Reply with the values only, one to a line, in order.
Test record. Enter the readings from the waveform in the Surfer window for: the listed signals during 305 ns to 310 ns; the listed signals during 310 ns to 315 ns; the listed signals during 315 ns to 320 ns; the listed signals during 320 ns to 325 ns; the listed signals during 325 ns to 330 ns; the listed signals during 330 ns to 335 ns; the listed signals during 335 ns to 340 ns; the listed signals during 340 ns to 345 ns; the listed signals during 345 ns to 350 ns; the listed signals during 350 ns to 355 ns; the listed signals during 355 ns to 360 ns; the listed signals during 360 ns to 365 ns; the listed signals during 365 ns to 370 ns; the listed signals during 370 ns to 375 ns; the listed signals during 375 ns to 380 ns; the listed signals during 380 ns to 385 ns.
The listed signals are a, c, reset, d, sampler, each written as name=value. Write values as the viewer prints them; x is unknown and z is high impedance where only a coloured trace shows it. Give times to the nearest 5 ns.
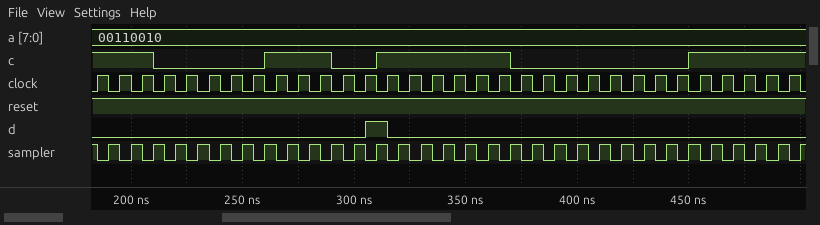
a=00110010, c=0, reset=1, d=1, sampler=0
a=00110010, c=1, reset=1, d=1, sampler=1
a=00110010, c=1, reset=1, d=0, sampler=0
a=00110010, c=1, reset=1, d=0, sampler=1
a=00110010, c=1, reset=1, d=0, sampler=0
a=00110010, c=1, reset=1, d=0, sampler=1
a=00110010, c=1, reset=1, d=0, sampler=0
a=00110010, c=1, reset=1, d=0, sampler=1
a=00110010, c=1, reset=1, d=0, sampler=0
a=00110010, c=1, reset=1, d=0, sampler=1
a=00110010, c=1, reset=1, d=0, sampler=0
a=00110010, c=1, reset=1, d=0, sampler=1
a=00110010, c=1, reset=1, d=0, sampler=0
a=00110010, c=0, reset=1, d=0, sampler=1
a=00110010, c=0, reset=1, d=0, sampler=0
a=00110010, c=0, reset=1, d=0, sampler=1
